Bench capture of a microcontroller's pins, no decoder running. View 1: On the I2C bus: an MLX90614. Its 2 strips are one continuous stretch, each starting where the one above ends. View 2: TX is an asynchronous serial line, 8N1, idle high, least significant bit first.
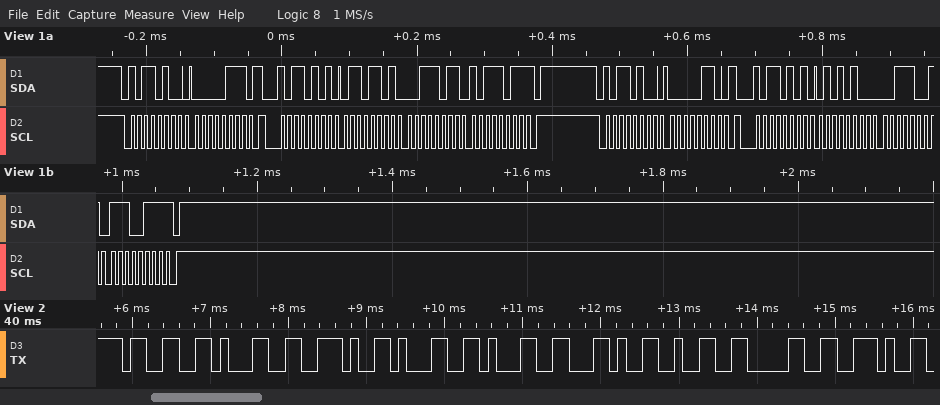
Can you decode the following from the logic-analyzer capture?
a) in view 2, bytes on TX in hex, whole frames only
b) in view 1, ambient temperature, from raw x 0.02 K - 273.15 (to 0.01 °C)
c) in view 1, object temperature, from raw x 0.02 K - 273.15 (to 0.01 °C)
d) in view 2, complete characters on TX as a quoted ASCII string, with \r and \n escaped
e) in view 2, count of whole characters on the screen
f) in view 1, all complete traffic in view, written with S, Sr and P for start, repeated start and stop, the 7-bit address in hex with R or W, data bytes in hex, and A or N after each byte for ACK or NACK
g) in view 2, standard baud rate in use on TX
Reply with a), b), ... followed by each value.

a) 33 31 2E 31 31 2C 32 30 2E
b) 20.37 °C
c) 31.11 °C
d) "31.11,20."
e) 9
f) S 5AW A 07 A Sr 5AR A 6D A 3B A BB N P S 5AW A 06 A Sr 5AR A 54 A 39 A E7 N P
g) 9600 baud
